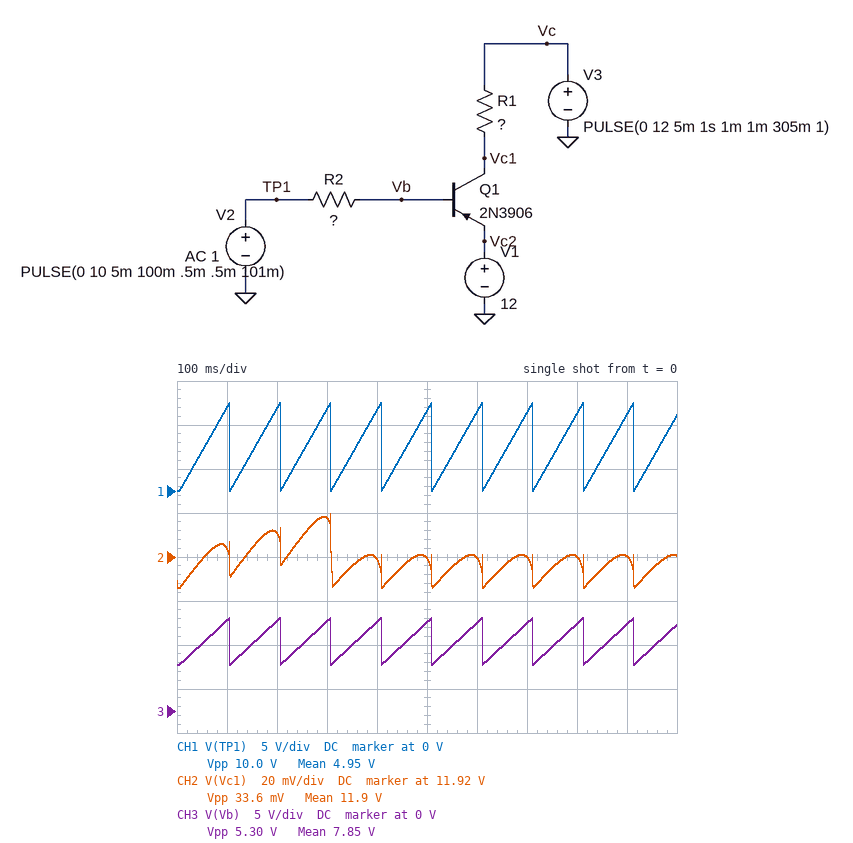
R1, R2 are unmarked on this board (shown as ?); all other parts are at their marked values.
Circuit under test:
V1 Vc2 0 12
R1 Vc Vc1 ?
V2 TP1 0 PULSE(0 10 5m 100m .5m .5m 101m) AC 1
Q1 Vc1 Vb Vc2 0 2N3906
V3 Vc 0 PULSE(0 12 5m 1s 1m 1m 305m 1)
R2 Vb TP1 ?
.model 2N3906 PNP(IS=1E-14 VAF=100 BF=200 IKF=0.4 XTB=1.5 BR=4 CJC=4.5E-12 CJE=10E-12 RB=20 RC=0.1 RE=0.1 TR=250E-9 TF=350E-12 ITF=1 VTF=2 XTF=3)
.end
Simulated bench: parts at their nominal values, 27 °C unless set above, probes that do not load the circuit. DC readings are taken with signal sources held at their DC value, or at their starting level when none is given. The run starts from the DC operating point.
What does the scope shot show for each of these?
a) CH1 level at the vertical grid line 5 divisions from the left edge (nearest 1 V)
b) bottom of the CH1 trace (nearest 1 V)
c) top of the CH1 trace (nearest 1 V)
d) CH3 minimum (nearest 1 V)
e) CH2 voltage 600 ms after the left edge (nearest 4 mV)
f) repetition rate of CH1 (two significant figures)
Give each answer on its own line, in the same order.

9 V
0 V
10 V
5 V
11.920 V
9.9 Hz
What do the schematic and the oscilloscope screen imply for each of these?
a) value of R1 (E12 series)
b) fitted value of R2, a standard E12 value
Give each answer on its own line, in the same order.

56 Ω
18 Ω
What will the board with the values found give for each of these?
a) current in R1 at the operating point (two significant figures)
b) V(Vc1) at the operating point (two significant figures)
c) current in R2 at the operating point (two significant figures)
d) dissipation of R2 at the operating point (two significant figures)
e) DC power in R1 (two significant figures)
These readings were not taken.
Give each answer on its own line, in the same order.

210 mA
12 V
290 mA
1.5 W
2.5 W
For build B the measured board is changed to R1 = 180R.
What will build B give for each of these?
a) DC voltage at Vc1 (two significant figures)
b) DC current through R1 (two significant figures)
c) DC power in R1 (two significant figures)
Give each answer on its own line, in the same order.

12 V
66 mA
790 mW
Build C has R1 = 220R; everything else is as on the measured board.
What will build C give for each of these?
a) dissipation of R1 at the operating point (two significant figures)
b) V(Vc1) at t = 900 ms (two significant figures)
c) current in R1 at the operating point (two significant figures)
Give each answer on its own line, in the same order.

650 mW
12 V
54 mA
